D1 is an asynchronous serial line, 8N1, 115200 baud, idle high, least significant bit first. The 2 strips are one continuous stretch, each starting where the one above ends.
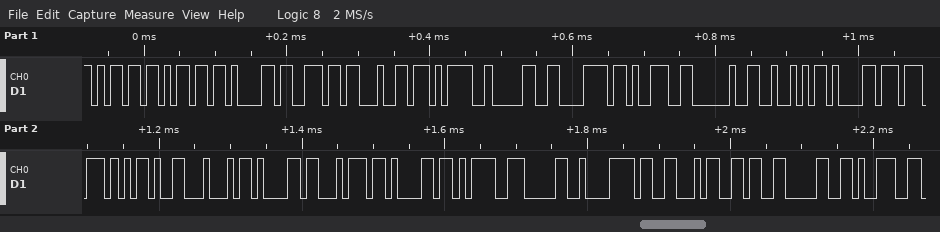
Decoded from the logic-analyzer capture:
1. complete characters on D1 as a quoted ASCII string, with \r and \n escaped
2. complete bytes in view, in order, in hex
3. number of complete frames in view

"mmand=0x9 Raw-Data=0xF609"
6D 6D 61 6E 64 3D 30 78 39 20 52 61 77 2D 44 61 74 61 3D 30 78 46 36 30 39
25
